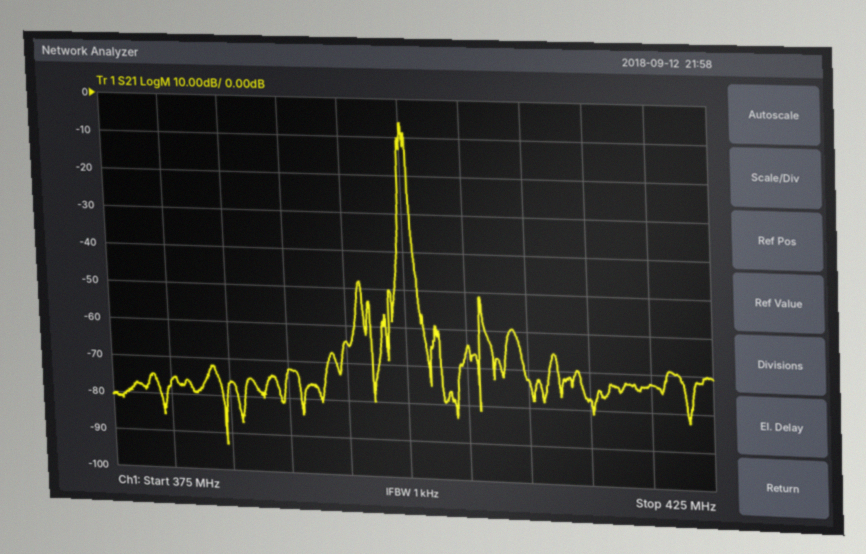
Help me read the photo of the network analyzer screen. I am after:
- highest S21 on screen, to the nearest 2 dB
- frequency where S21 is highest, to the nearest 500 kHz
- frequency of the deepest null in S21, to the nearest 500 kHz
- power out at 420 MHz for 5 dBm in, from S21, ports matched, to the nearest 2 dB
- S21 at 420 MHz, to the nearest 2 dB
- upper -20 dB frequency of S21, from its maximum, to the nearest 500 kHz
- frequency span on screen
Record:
-6 dB
400.0 MHz
384.5 MHz
-68 dBm
-72 dB
400.5 MHz
50 MHz
